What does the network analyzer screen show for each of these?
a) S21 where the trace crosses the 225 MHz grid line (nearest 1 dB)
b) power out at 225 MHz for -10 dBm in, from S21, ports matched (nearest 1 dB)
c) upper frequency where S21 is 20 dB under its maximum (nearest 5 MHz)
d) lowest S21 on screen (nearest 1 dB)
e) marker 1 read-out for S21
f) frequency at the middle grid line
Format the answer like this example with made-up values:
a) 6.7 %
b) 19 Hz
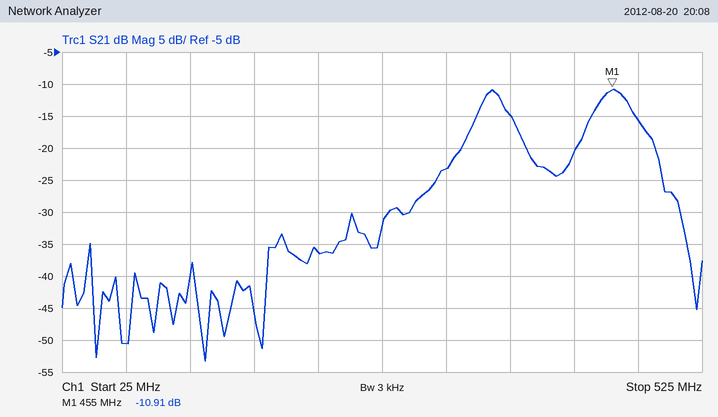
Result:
a) -36 dB
b) -46 dBm
c) 510 MHz
d) -53 dB
e) -10.91 dB
f) 275 MHz
